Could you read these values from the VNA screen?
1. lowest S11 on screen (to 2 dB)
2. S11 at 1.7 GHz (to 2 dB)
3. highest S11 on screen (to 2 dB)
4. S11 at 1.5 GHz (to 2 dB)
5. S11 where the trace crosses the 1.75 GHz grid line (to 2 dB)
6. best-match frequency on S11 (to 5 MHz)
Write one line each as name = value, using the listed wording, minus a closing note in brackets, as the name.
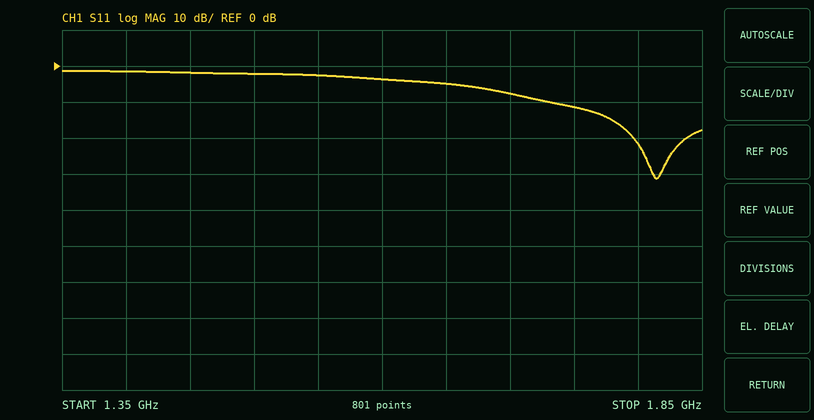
lowest S11 on screen = -32 dB
S11 at 1.7 GHz = -8 dB
highest S11 on screen = -2 dB
S11 at 1.5 GHz = -2 dB
S11 where the trace crosses the 1.75 GHz grid line = -12 dB
best-match frequency on S11 = 1.815 GHz
